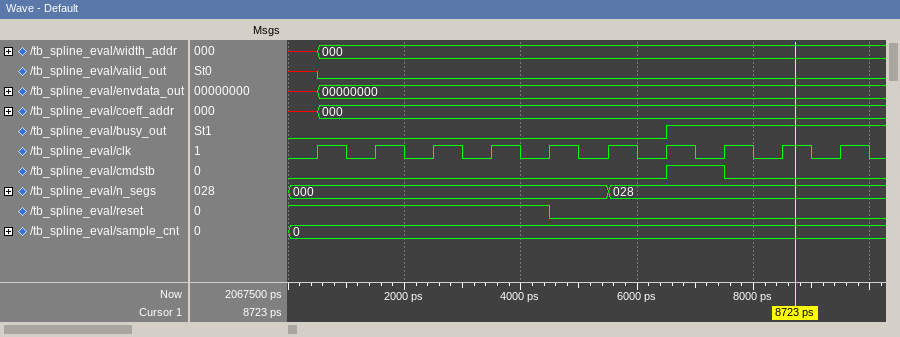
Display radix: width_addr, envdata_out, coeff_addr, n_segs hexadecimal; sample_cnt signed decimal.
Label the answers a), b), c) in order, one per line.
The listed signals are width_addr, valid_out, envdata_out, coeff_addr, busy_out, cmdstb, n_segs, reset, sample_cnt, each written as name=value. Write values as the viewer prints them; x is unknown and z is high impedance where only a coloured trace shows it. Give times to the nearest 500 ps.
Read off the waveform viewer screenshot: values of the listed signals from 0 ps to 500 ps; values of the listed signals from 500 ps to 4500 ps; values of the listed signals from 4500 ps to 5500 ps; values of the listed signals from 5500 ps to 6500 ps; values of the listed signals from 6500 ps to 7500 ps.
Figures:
a) width_addr=x, valid_out=x, envdata_out=x, coeff_addr=x, busy_out=0, cmdstb=0, n_segs=000, reset=1, sample_cnt=0
b) width_addr=000, valid_out=0, envdata_out=00000000, coeff_addr=000, busy_out=0, cmdstb=0, n_segs=000, reset=1, sample_cnt=0
c) width_addr=000, valid_out=0, envdata_out=00000000, coeff_addr=000, busy_out=0, cmdstb=0, n_segs=000, reset=0, sample_cnt=0
d) width_addr=000, valid_out=0, envdata_out=00000000, coeff_addr=000, busy_out=0, cmdstb=0, n_segs=028, reset=0, sample_cnt=0
e) width_addr=000, valid_out=0, envdata_out=00000000, coeff_addr=000, busy_out=1, cmdstb=1, n_segs=028, reset=0, sample_cnt=0
